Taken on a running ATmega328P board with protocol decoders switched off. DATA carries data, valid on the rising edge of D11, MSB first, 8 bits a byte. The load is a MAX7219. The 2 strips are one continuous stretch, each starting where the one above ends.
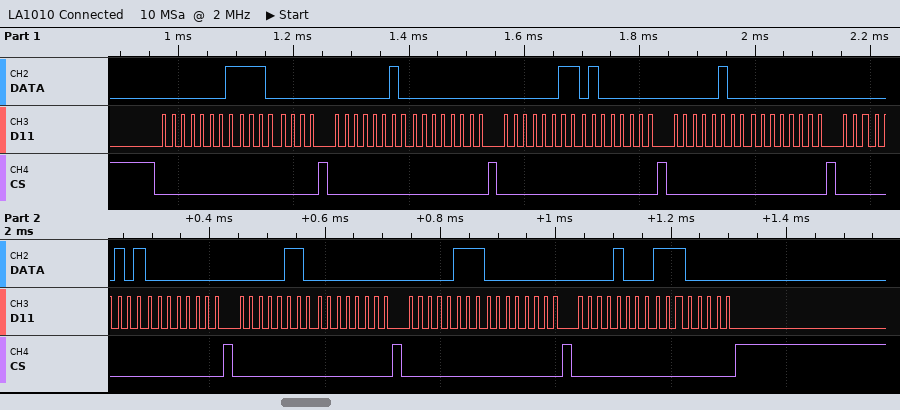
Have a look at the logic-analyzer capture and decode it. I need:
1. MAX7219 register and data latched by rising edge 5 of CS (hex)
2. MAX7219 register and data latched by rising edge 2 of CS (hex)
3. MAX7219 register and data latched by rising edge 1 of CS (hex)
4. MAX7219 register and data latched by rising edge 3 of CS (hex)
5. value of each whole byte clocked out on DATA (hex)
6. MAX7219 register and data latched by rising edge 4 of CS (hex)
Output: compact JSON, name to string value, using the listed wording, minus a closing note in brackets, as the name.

{"MAX7219 register and data latched by rising edge 5 of CS": "register 0x5, data 0x00", "MAX7219 register and data latched by rising edge 2 of CS": "register 0x2, data 0x00", "MAX7219 register and data latched by rising edge 1 of CS": "register 0x1, data 0xE0", "MAX7219 register and data latched by rising edge 3 of CS": "register 0x3, data 0x40", "value of each whole byte clocked out on DATA": "01 E0 02 00 03 40 04 00 05 00 06 00 07 00 08 E0", "MAX7219 register and data latched by rising edge 4 of CS": "register 0x4, data 0x00"}
